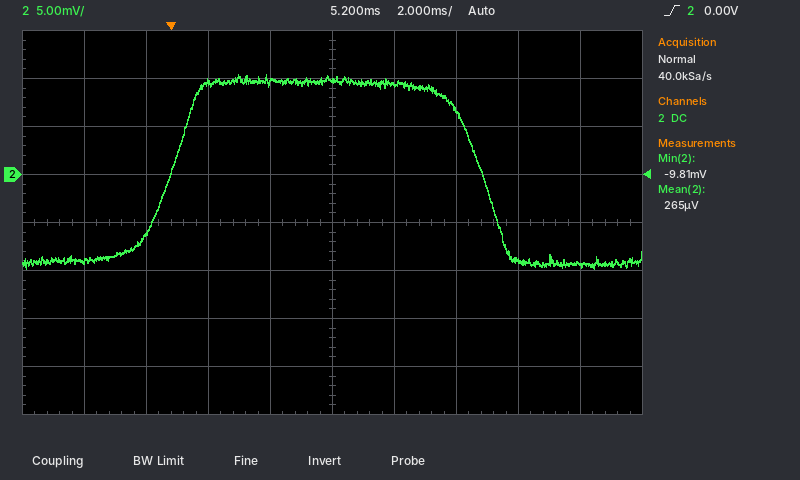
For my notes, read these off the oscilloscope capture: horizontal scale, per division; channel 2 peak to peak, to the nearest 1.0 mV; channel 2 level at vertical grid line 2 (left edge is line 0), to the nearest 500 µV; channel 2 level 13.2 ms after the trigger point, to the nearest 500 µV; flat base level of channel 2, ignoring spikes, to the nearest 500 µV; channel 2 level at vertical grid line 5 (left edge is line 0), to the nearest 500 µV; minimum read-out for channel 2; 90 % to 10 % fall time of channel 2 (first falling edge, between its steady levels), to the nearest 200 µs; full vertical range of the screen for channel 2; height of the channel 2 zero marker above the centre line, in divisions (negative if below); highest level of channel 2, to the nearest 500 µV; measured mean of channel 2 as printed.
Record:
2 ms
20.0 mV
-6.0 mV
-9.5 mV
-9.0 mV
10.0 mV
-9.81 mV
1.8 ms
40 mV
+1.0 div
10.5 mV
265 µV
